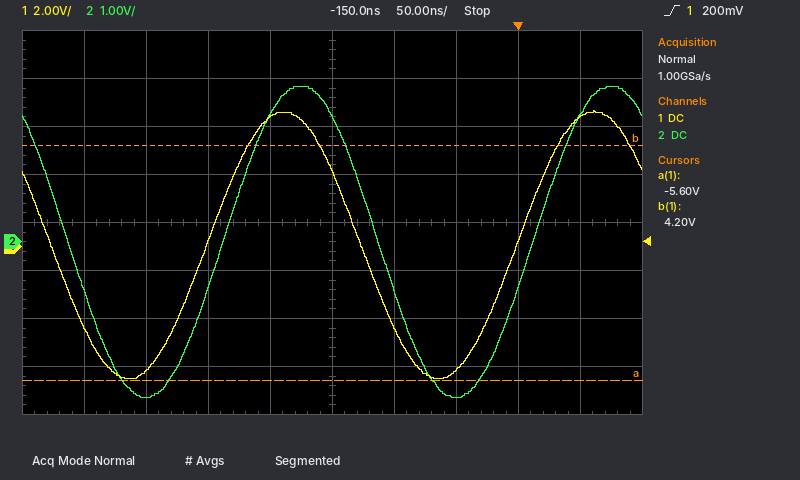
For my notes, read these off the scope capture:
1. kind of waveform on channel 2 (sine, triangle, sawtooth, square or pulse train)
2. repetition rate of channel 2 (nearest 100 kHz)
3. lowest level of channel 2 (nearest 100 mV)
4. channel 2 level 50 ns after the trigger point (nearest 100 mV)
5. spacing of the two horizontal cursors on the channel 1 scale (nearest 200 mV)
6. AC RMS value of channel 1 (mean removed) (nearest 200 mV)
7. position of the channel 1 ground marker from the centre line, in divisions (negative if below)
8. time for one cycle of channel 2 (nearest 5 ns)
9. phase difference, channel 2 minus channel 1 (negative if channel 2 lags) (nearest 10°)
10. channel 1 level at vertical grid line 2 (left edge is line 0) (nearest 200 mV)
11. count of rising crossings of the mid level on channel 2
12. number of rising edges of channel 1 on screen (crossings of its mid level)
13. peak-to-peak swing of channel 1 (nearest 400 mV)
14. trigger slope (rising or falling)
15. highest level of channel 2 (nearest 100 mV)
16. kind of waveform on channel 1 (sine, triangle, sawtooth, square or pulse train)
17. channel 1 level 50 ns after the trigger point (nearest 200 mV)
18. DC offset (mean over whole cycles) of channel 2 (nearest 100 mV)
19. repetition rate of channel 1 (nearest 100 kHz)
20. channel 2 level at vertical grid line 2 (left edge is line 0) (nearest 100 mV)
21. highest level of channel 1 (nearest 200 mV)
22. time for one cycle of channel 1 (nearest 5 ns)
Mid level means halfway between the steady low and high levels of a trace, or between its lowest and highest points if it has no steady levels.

sine
4.0 MHz
-3.2 V
2.6 V
9.8 V
4.0 V
-0.5 div
250 ns
-20°
-5.2 V
2
2
11.2 V
rising
3.2 V
sine
5.4 V
0.0 V
4.0 MHz
-3.2 V
5.6 V
250 ns
